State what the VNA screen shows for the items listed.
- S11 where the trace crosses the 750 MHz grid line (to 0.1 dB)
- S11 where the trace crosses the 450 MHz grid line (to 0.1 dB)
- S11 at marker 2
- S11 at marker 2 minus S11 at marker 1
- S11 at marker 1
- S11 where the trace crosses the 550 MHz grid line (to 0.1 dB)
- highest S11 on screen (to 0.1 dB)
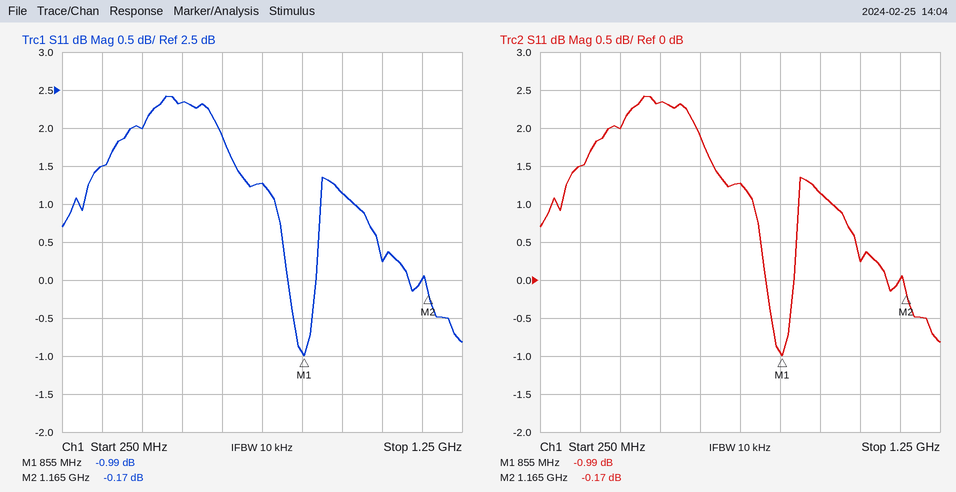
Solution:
1.3 dB
2.0 dB
-0.17 dB
0.82 dB
-0.99 dB
2.3 dB
2.4 dB
